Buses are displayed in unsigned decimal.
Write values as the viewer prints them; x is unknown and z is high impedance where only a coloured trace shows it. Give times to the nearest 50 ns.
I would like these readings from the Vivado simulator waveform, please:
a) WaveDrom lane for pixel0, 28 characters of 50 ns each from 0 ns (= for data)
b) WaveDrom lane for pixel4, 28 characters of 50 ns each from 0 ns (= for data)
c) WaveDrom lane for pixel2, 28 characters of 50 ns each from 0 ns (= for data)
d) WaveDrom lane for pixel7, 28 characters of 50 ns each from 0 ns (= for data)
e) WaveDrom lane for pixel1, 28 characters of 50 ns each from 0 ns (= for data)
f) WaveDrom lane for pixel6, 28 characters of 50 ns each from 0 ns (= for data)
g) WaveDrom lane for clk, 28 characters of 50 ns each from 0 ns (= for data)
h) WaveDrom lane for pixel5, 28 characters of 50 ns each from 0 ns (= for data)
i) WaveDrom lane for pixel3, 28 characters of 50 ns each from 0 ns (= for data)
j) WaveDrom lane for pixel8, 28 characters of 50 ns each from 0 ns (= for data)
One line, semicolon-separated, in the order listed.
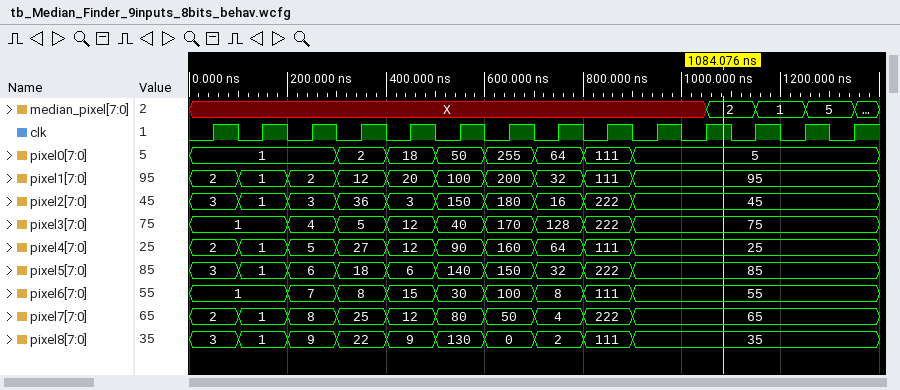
{name: 'pixel0', wave: '=.....=.=.=.=.=.=.=.........', data: '1 2 18 50 255 64 111 5'}; {name: 'pixel4', wave: '=.=.=.=.=.=.=.=.=.=.........', data: '2 1 5 27 12 90 160 64 111 25'}; {name: 'pixel2', wave: '=.=.=.=.=.=.=.=.=.=.........', data: '3 1 3 36 3 150 180 16 222 45'}; {name: 'pixel7', wave: '=.=.=.=.=.=.=.=.=.=.........', data: '2 1 8 25 12 80 50 4 222 65'}; {name: 'pixel1', wave: '=.=.=.=.=.=.=.=.=.=.........', data: '2 1 2 12 20 100 200 32 111 95'}; {name: 'pixel6', wave: '=...=.=.=.=.=.=.=.=.........', data: '1 7 8 15 30 100 8 111 55'}; {name: 'clk', wave: '0101010101010101010101010101'}; {name: 'pixel5', wave: '=.=.=.=.=.=.=.=.=.=.........', data: '3 1 6 18 6 140 150 32 222 85'}; {name: 'pixel3', wave: '=...=.=.=.=.=.=.=.=.........', data: '1 4 5 12 40 170 128 222 75'}; {name: 'pixel8', wave: '=.=.=.=.=.=.=.=.=.=.........', data: '3 1 9 22 9 130 0 2 111 35'}
